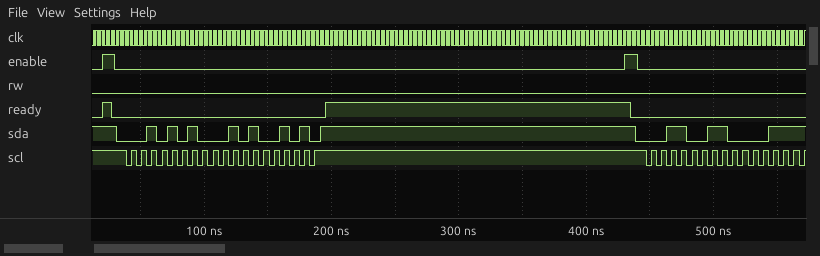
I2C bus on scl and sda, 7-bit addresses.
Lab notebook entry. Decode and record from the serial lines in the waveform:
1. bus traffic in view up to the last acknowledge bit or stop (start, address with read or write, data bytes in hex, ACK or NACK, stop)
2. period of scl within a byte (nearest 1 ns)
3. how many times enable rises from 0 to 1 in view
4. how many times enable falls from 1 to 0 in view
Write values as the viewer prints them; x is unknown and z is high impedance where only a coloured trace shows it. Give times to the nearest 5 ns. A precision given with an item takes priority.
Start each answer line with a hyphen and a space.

- start, address 15 write ACK, 52 NACK, stop, start, address 19 read ACK
- 8 ns
- 2
- 2
